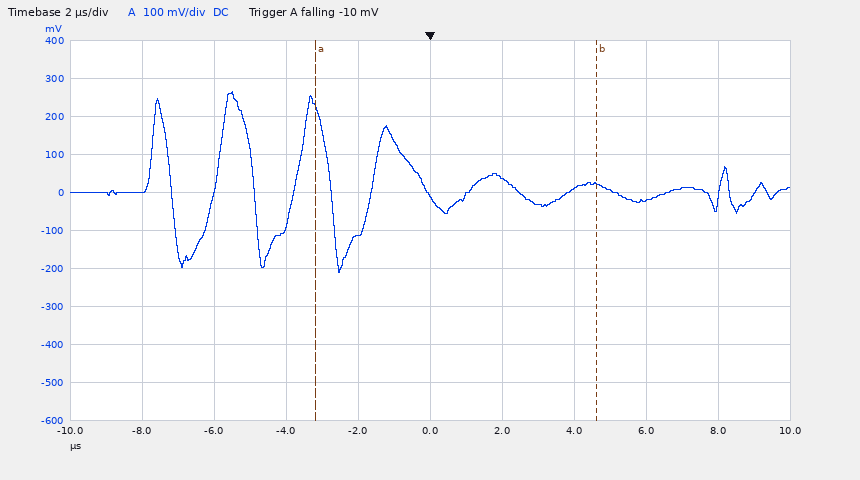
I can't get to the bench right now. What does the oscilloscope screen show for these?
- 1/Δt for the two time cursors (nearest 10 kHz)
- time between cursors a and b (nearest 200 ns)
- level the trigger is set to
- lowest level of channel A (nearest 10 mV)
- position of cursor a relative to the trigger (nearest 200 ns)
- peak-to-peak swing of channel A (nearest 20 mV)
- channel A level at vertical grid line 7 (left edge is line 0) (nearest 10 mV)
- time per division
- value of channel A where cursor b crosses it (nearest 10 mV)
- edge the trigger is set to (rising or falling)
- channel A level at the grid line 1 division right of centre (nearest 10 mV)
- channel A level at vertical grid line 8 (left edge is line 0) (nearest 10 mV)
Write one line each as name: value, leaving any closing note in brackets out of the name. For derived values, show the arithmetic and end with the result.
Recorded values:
1/Δt for the two time cursors: 1 / 7.8 µs ≈ 130 kHz
time between cursors a and b: 7.8 µs
level the trigger is set to: -10 mV
lowest level of channel A: -210 mV
position of cursor a relative to the trigger: -3.2 µs
peak-to-peak swing of channel A: 480 mV
channel A level at vertical grid line 7 (left edge is line 0): 10 mV
time per division: 2 µs
value of channel A where cursor b crosses it: 20 mV
edge the trigger is set to: falling
channel A level at the grid line 1 division right of centre: 40 mV
channel A level at vertical grid line 8 (left edge is line 0): -20 mV
